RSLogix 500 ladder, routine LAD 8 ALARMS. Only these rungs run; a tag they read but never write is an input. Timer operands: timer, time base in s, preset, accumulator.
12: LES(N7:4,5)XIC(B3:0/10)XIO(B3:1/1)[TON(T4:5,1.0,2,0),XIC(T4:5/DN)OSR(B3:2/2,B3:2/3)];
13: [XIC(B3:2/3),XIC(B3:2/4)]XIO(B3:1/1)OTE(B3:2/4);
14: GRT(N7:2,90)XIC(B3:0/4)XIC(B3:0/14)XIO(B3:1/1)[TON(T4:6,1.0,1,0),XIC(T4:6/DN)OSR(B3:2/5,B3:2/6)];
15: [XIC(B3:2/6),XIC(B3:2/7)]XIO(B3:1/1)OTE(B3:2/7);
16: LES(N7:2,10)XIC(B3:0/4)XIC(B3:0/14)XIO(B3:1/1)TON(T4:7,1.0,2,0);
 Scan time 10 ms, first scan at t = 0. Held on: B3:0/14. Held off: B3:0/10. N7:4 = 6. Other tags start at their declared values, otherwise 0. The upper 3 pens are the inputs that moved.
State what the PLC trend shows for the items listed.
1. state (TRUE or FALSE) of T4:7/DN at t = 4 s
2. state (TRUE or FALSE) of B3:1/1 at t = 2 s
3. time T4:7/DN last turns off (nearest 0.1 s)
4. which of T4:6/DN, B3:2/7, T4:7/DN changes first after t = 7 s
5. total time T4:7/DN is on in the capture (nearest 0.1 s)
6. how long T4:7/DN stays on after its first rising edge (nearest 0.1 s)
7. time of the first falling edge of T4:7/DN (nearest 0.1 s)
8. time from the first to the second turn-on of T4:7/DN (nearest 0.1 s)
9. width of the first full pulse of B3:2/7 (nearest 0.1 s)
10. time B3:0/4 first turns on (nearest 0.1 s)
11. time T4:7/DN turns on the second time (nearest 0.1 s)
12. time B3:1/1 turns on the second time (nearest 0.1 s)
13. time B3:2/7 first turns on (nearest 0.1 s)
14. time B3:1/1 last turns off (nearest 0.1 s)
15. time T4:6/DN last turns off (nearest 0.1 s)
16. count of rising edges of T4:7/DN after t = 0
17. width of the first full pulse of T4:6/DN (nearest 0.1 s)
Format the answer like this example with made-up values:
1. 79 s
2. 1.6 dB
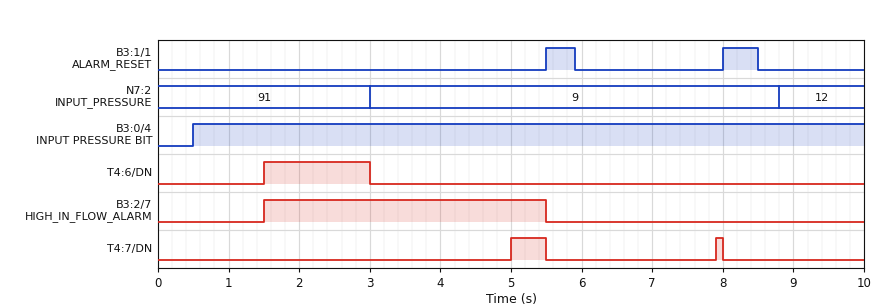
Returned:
1. FALSE
2. FALSE
3. 8.0 s
4. T4:7/DN
5. 0.6 s
6. 0.5 s
7. 5.5 s
8. 2.9 s
9. 4.0 s
10. 0.5 s
11. 7.9 s
12. 8.0 s
13. 1.5 s
14. 8.5 s
15. 3.0 s
16. 2
17. 1.5 s
